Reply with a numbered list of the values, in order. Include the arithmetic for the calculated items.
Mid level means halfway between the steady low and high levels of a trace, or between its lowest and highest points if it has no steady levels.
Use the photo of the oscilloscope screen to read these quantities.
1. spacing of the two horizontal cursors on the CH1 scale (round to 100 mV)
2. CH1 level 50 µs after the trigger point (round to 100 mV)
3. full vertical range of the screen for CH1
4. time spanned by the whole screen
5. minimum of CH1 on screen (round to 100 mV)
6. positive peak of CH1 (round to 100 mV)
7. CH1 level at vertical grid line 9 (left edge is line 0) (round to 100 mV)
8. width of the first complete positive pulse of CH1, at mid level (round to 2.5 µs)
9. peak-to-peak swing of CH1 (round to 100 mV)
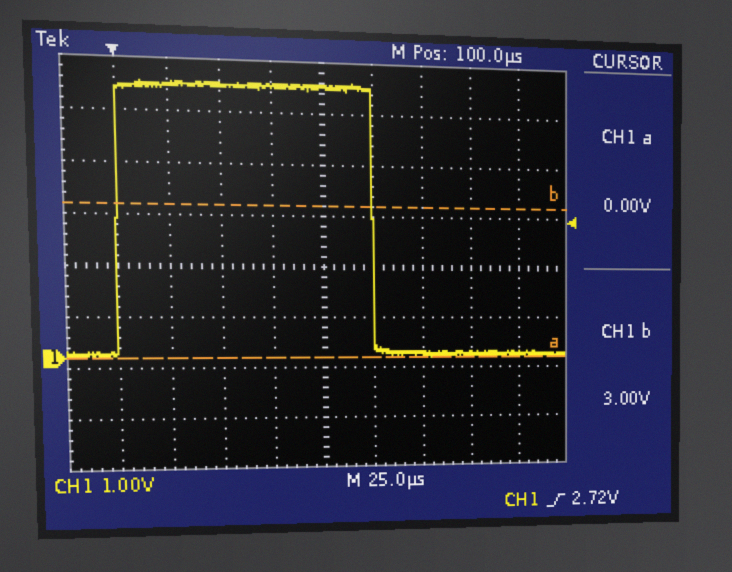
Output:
1. 3.0 V
2. 5.3 V
3. 8 V
4. 250 µs
5. 0.0 V
6. 5.4 V
7. 100 mV
8. 125.0 µs
9. 5.4 V − (0.0 V) = 5.4 V
